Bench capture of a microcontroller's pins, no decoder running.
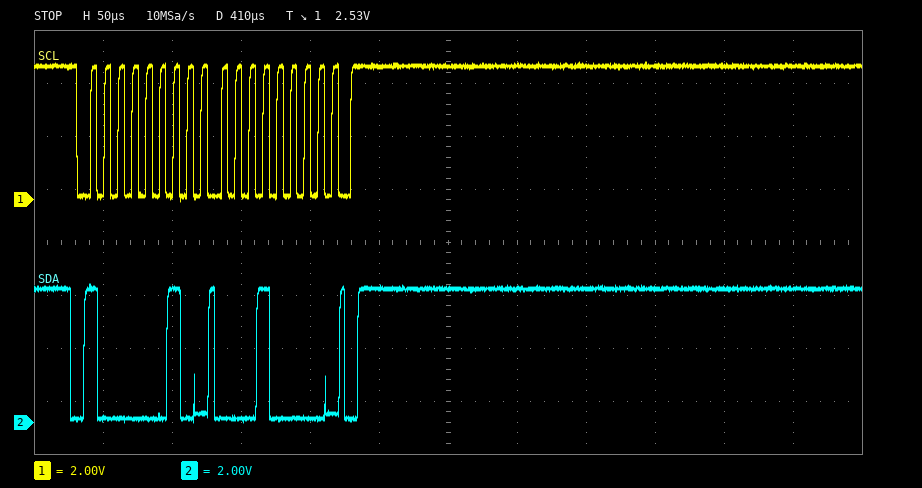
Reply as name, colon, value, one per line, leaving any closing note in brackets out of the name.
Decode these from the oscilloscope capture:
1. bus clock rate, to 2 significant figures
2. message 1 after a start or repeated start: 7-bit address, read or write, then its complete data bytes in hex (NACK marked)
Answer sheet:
bus clock rate, to 2 significant figures: 100 kHz
message 1 after a start or repeated start: 7-bit address, read or write, then its complete data bytes in hex: 0x41 write: 10
